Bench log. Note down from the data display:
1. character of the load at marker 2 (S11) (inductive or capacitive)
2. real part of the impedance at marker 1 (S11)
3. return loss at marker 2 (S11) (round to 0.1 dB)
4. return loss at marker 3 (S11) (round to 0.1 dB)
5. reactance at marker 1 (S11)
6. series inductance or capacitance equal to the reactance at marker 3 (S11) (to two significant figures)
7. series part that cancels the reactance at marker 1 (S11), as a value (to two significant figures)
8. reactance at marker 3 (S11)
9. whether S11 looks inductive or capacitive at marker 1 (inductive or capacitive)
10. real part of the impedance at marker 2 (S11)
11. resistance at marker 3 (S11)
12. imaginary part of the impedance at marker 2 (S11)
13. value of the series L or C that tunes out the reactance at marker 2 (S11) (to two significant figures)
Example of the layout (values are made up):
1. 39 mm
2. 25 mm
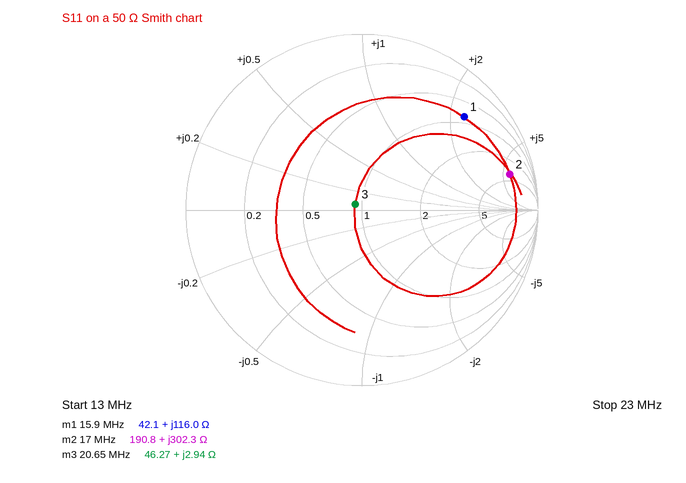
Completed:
1. inductive
2. 42.1 Ω
3. 1.3 dB
4. 26.1 dB
5. +116.0 Ω
6. 23 nH
7. 86 pF
8. +2.94 Ω
9. inductive
10. 190.8 Ω
11. 46.27 Ω
12. +302.3 Ω
13. 31 pF
